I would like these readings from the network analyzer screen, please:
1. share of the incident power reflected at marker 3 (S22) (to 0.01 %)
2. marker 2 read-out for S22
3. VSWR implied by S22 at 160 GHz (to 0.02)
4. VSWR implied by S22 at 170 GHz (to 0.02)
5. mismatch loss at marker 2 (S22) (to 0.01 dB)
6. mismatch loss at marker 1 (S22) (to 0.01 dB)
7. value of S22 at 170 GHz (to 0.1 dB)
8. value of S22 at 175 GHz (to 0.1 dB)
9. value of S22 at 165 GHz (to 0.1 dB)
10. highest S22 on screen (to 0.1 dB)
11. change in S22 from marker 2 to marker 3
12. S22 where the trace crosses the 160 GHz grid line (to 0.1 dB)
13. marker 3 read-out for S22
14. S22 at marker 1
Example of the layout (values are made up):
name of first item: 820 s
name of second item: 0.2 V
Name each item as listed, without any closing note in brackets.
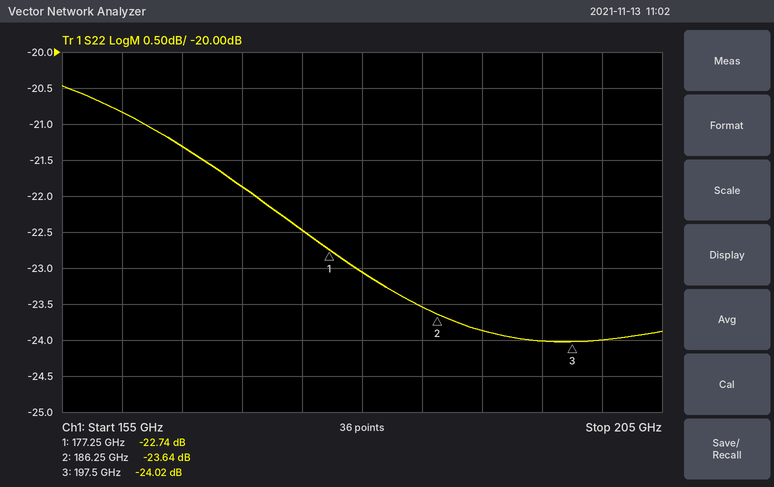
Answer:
share of the incident power reflected at marker 3 (S22): 0.40 %
marker 2 read-out for S22: -23.64 dB
VSWR implied by S22 at 160 GHz: 1.20
VSWR implied by S22 at 170 GHz: 1.18
mismatch loss at marker 2 (S22): 0.02 dB
mismatch loss at marker 1 (S22): 0.02 dB
value of S22 at 170 GHz: -21.9 dB
value of S22 at 175 GHz: -22.5 dB
value of S22 at 165 GHz: -21.3 dB
highest S22 on screen: -20.5 dB
change in S22 from marker 2 to marker 3: -0.38 dB
S22 where the trace crosses the 160 GHz grid line: -20.8 dB
marker 3 read-out for S22: -24.02 dB
S22 at marker 1: -22.74 dB
